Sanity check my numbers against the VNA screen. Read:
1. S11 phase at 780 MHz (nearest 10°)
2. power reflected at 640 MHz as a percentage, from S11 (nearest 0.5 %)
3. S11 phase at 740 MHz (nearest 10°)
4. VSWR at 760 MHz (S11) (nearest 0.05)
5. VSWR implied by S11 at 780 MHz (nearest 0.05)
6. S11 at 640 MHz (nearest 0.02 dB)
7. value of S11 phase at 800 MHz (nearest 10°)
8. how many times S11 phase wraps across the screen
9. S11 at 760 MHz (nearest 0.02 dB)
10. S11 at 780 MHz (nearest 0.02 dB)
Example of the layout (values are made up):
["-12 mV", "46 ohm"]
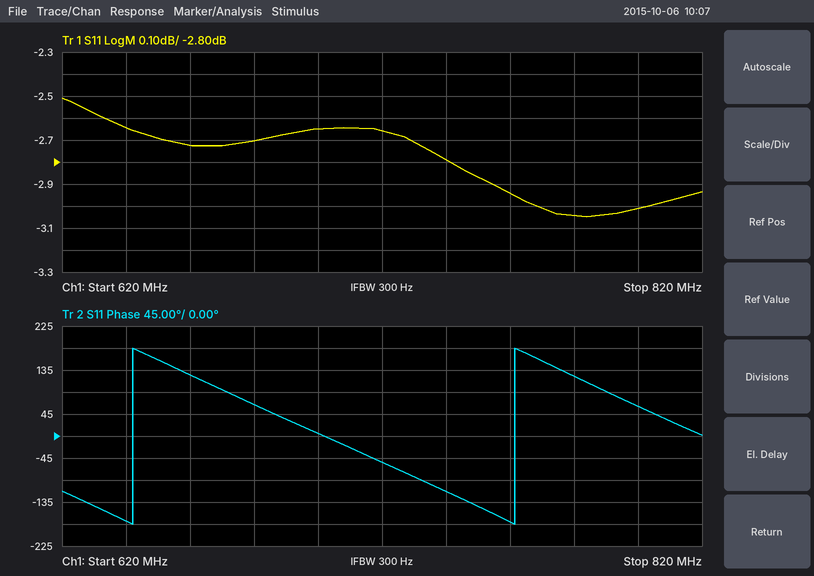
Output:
["120°", "54.5 %", "-110°", "5.95", "5.75", "-2.64 dB", "60°", "2", "-2.94 dB", "-3.04 dB"]
